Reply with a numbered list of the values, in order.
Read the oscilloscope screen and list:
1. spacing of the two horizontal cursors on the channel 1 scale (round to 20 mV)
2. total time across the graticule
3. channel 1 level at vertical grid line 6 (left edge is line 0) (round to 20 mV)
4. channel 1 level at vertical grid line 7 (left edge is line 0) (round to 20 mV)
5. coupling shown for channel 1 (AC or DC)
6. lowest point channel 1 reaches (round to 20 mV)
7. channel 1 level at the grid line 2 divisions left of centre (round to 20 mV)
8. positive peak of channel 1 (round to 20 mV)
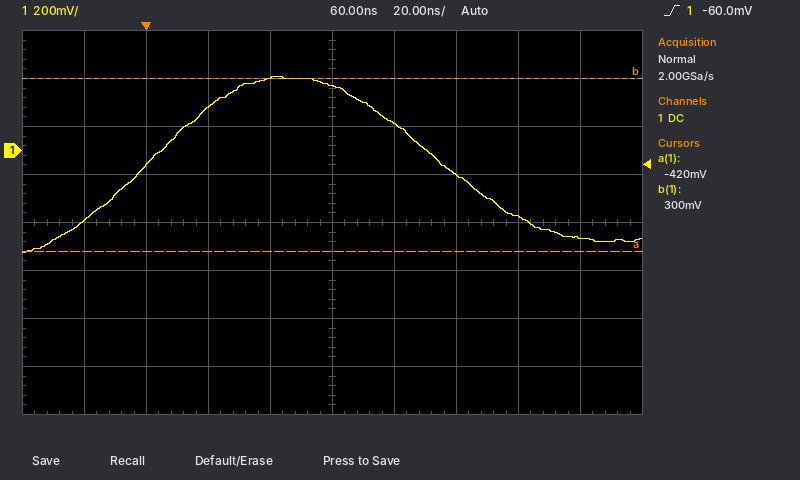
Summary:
1. 720 mV
2. 200 ns
3. 120 mV
4. -100 mV
5. DC
6. -420 mV
7. 180 mV
8. 300 mV
